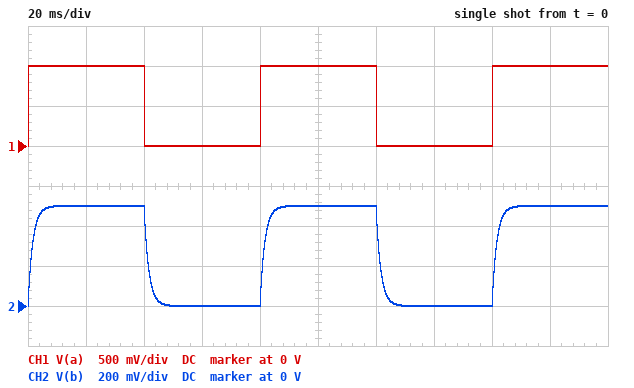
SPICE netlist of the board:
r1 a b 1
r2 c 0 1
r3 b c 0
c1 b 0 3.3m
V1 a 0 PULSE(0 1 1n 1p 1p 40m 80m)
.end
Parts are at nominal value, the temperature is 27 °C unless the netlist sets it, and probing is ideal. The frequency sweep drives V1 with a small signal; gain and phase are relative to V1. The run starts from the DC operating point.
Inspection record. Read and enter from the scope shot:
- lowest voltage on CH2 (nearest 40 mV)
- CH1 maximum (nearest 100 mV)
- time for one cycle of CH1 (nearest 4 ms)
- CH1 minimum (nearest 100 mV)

0 V
1.0 V
80 ms
0 V
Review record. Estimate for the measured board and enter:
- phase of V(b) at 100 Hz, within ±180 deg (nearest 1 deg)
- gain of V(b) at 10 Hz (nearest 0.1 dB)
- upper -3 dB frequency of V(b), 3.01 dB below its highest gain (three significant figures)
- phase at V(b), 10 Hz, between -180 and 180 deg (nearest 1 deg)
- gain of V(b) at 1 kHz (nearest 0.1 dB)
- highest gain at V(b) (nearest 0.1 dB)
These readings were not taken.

-46 deg
-6.1 dB
96.5 Hz
-6 deg
-26.4 dB
-6.0 dB
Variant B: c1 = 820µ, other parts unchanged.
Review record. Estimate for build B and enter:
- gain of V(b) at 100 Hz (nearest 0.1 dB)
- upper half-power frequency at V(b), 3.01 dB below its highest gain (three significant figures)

-6.3 dB
388 Hz
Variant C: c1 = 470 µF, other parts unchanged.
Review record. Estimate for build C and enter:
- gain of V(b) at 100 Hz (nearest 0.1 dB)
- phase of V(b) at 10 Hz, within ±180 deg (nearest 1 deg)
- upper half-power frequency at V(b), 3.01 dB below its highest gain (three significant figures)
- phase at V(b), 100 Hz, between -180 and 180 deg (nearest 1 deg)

-6.1 dB
-1 deg
677 Hz
-8 deg
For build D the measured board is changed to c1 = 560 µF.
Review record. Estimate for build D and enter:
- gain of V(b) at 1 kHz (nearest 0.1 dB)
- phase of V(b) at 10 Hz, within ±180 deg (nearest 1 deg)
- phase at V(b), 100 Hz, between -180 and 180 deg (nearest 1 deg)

-12.1 dB
-1 deg
-10 deg
